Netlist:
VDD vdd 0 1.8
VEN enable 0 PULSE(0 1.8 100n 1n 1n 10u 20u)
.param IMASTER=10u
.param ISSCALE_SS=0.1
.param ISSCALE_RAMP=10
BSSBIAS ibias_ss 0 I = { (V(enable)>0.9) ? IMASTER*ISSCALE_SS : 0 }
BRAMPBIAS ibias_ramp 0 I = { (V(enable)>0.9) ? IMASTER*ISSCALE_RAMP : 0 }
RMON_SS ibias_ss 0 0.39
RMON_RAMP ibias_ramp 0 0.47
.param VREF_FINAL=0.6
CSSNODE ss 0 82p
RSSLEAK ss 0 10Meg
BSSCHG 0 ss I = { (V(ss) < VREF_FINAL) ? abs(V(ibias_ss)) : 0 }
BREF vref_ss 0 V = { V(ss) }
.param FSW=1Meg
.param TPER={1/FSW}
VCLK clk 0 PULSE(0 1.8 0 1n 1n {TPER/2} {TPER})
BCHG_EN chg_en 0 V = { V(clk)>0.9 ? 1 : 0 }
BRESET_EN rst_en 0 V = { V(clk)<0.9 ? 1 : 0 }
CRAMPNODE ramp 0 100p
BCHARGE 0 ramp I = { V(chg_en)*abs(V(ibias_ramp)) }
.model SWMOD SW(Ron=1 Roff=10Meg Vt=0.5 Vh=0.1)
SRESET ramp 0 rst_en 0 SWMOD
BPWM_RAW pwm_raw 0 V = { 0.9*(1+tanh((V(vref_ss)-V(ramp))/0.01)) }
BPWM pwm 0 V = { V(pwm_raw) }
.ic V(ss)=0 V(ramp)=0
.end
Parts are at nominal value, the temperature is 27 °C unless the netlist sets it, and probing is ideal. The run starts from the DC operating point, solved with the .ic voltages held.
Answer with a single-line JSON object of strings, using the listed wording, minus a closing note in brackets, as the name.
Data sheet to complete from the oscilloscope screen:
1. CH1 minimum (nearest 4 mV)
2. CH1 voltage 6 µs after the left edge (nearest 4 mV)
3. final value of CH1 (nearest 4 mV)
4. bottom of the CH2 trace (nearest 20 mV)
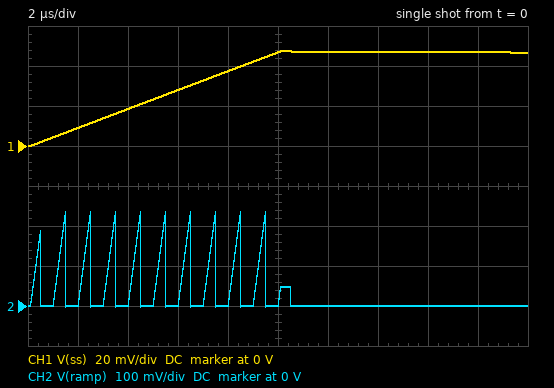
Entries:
{"CH1 minimum": "0 V", "CH1 voltage 6 µs after the left edge": "28 mV", "final value of CH1": "48 mV", "bottom of the CH2 trace": "0 V"}
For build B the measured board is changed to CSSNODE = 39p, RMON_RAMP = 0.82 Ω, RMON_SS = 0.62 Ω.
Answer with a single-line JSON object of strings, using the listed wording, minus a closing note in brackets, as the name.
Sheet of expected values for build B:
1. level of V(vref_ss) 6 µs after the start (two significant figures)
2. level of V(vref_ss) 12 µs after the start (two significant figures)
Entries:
{"level of V(vref_ss) 6 µs after the start": "93 mV", "level of V(vref_ss) 12 µs after the start": "160 mV"}
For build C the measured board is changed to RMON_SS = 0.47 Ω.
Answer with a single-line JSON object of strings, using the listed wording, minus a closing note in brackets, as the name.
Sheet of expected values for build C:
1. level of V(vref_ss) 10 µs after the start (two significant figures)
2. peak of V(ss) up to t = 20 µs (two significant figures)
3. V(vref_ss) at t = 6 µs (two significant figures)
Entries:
{"level of V(vref_ss) 10 µs after the start": "56 mV", "peak of V(ss) up to t = 20 µs": "57 mV", "V(vref_ss) at t = 6 µs": "34 mV"}
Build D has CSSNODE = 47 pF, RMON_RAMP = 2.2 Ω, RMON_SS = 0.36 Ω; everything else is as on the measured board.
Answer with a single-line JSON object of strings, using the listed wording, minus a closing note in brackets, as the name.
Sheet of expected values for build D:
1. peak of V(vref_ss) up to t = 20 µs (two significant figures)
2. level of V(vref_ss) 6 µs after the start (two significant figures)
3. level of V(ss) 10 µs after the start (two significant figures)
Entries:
{"peak of V(vref_ss) up to t = 20 µs": "76 mV", "level of V(vref_ss) 6 µs after the start": "45 mV", "level of V(ss) 10 µs after the start": "75 mV"}
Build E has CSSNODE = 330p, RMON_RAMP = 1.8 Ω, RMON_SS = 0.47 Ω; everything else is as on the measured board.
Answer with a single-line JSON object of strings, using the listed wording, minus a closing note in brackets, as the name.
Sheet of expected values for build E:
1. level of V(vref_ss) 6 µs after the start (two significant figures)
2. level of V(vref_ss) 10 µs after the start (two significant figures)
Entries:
{"level of V(vref_ss) 6 µs after the start": "8.4 mV", "level of V(vref_ss) 10 µs after the start": "14 mV"}
